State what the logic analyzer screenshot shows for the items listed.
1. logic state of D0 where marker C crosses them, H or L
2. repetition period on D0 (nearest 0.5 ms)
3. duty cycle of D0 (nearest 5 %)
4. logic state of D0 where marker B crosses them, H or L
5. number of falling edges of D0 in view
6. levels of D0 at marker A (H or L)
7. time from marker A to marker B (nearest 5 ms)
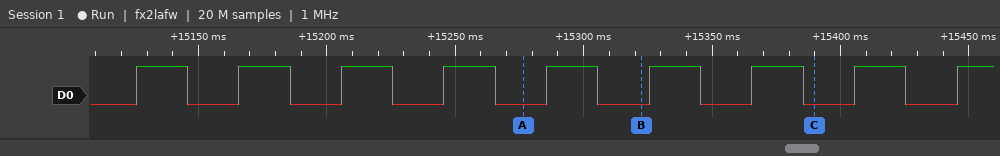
D0=L
40 ms
50 %
D0=L
8
D0=L
45 ms
